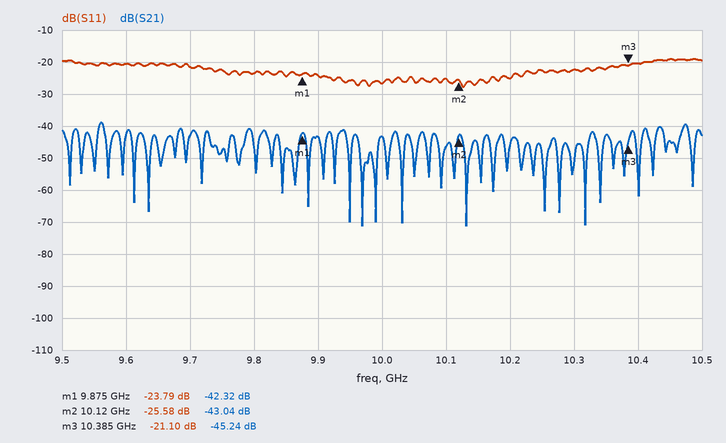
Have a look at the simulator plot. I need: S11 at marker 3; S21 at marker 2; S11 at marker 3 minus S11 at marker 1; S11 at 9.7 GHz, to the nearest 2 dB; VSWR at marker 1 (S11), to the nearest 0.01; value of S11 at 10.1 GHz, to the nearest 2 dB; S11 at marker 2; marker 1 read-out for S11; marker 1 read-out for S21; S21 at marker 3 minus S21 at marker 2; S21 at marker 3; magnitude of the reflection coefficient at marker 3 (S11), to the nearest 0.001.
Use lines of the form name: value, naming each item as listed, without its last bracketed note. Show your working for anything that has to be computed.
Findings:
S11 at marker 3: -21.10 dB
S21 at marker 2: -43.04 dB
S11 at marker 3 minus S11 at marker 1: -21.1 − (-23.79) = 2.69 dB
S11 at 9.7 GHz, to the nearest 2 dB: -22 dB
VSWR at marker 1 (S11), to the nearest 0.01: (1 + 0.0646)/(1 − 0.0646) ≈ 1.14
value of S11 at 10.1 GHz, to the nearest 2 dB: -26 dB
S11 at marker 2: -25.58 dB
marker 1 read-out for S11: -23.79 dB
marker 1 read-out for S21: -42.32 dB
S21 at marker 3 minus S21 at marker 2: -45.24 − (-43.04) = -2.20 dB
S21 at marker 3: -45.24 dB
magnitude of the reflection coefficient at marker 3 (S11), to the nearest 0.001: 10^(-21.1/20) ≈ 0.088
